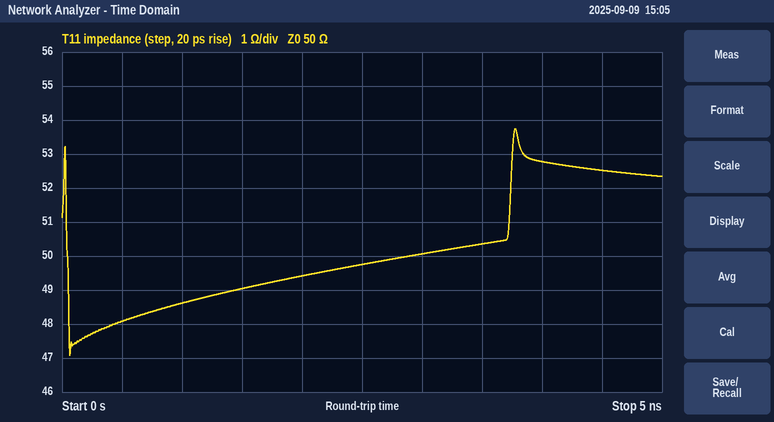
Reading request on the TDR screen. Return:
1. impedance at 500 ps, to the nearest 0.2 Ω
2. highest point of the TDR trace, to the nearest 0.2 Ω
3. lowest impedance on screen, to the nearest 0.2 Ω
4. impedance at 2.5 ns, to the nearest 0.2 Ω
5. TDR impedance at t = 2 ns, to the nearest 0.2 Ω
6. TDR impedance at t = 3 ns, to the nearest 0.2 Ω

48.0 Ω
53.8 Ω
47.0 Ω
49.8 Ω
49.4 Ω
50.0 Ω
